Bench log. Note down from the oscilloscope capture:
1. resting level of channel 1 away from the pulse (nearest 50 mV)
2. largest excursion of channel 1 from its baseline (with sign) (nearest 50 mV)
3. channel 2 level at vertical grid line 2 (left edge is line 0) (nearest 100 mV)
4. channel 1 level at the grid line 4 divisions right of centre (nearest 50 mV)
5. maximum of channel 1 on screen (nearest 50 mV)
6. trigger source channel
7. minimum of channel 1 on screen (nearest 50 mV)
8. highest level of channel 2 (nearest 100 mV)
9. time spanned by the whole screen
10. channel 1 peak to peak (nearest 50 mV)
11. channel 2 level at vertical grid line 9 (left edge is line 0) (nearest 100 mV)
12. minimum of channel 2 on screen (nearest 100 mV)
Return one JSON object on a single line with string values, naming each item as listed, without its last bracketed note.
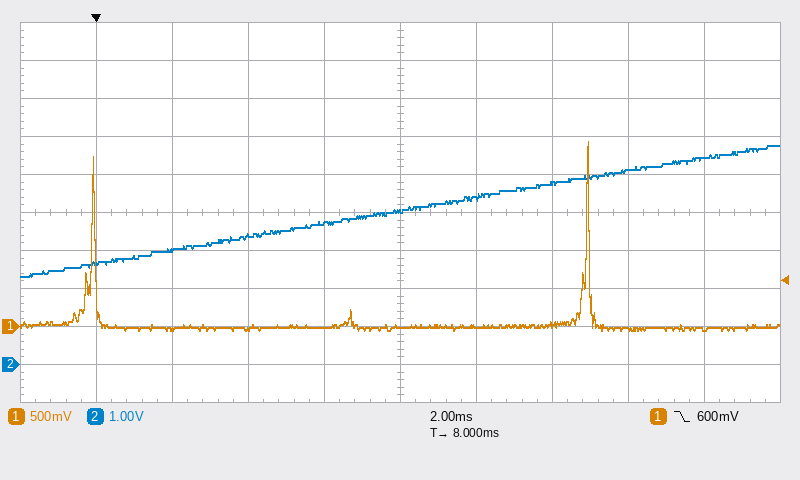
{"resting level of channel 1 away from the pulse": "0 mV", "largest excursion of channel 1 from its baseline (with sign)": "+2.45 V", "channel 2 level at vertical grid line 2 (left edge is line 0)": "3.0 V", "channel 1 level at the grid line 4 divisions right of centre": "-50 mV", "maximum of channel 1 on screen": "2.45 V", "trigger source channel": "channel 1", "minimum of channel 1 on screen": "-50 mV", "highest level of channel 2": "5.8 V", "time spanned by the whole screen": "20 ms", "channel 1 peak to peak": "2.50 V", "channel 2 level at vertical grid line 9 (left edge is line 0)": "5.4 V", "minimum of channel 2 on screen": "2.3 V"}
